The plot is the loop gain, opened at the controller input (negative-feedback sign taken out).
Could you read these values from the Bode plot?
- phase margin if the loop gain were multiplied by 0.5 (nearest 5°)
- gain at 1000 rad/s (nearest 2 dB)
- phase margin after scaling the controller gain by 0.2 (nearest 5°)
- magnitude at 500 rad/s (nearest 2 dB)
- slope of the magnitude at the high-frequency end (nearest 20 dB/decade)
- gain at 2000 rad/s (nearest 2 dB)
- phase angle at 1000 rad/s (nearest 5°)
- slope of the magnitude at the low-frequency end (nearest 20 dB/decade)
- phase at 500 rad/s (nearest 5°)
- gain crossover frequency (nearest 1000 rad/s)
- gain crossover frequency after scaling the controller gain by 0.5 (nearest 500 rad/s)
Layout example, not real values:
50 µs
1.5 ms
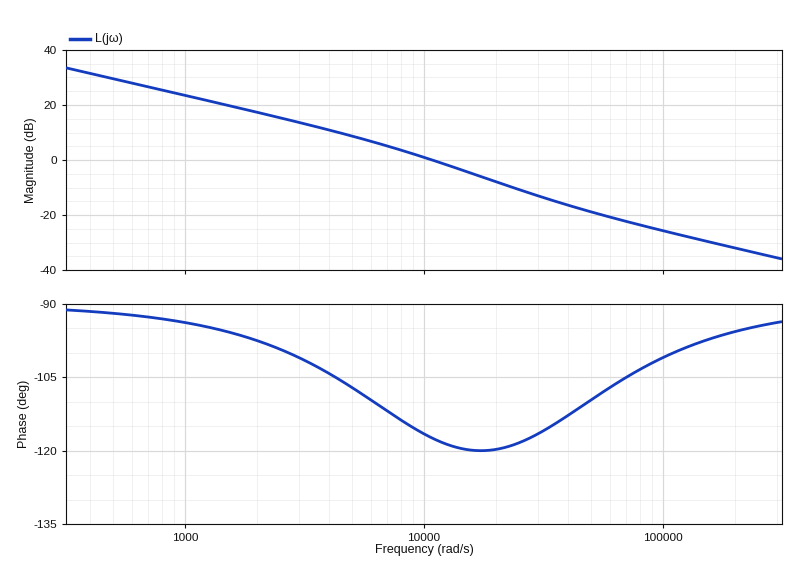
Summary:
70°
24 dB
80°
30 dB
-20 dB/decade
18 dB
-95°
-20 dB/decade
-90°
11000 rad/s
6500 rad/s
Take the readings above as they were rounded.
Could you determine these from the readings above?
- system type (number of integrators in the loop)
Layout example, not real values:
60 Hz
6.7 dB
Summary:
1
